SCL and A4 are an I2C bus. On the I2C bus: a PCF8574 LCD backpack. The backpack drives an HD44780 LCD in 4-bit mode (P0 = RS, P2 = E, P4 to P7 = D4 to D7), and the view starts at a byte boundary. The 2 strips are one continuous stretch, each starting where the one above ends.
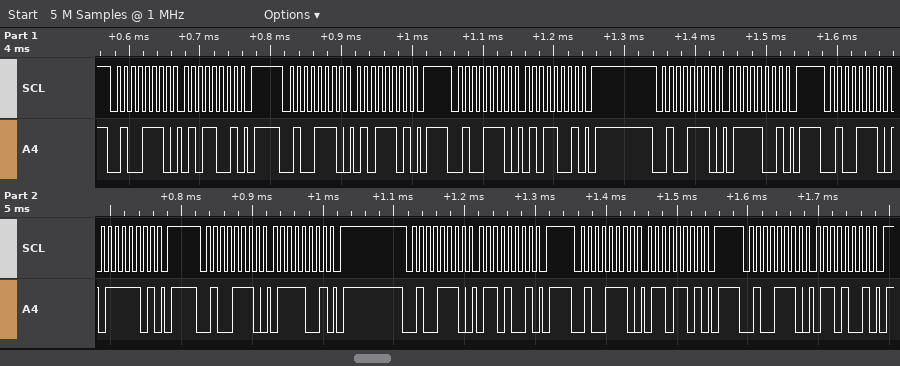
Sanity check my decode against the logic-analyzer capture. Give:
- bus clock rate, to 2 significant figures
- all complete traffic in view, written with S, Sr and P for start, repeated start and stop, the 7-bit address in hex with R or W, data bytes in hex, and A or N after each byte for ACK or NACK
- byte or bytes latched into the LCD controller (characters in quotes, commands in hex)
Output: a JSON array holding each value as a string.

["100 kHz", "S 27W A 59 A P S 27W A 5D A P S 27W A 59 A P S 27W A 79 A P S 27W A 7D A P S 27W A 79 A P S 27W A 69 A P S 27W A 6D A P S 27W A 69 A P", "'W'"]
